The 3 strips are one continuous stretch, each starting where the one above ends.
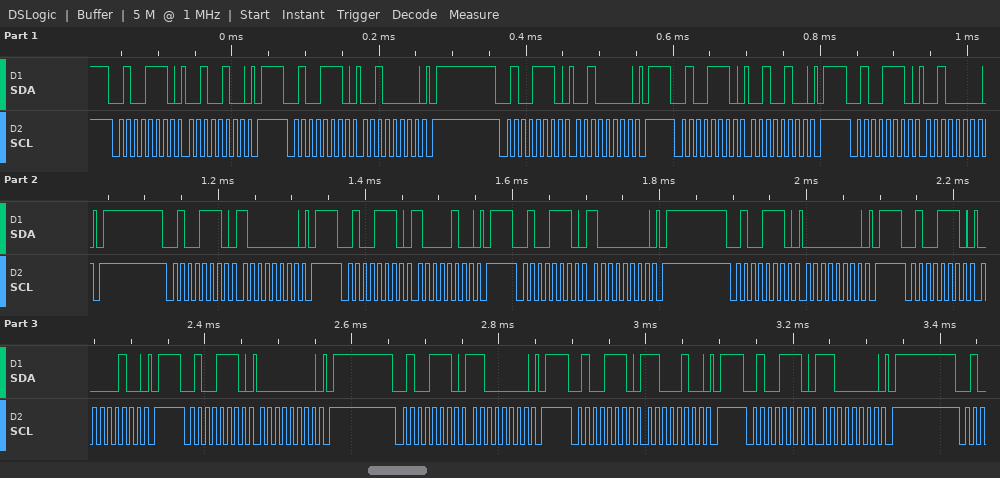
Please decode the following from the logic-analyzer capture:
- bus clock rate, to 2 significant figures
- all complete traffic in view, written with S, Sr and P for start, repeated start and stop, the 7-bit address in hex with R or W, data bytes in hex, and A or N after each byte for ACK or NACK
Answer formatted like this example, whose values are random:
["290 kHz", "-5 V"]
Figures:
["100 kHz", "S 27W A 24 A P S 27W A 20 A P S 27W A 20 A P S 27W A 24 A P S 27W A 20 A P S 27W A 80 A P S 27W A 84 A P S 27W A 80 A P S 27W A 00 A P S 27W A 04 A P S 27W A 00 A P S 27W A C0 A P S 27W A C4 A P S 27W A C0 A P"]
